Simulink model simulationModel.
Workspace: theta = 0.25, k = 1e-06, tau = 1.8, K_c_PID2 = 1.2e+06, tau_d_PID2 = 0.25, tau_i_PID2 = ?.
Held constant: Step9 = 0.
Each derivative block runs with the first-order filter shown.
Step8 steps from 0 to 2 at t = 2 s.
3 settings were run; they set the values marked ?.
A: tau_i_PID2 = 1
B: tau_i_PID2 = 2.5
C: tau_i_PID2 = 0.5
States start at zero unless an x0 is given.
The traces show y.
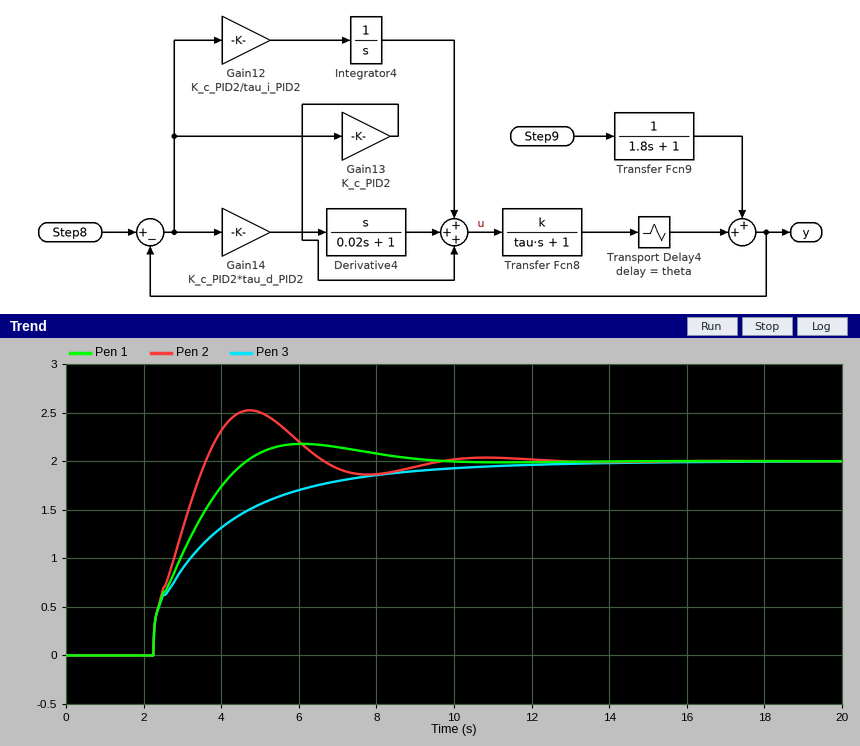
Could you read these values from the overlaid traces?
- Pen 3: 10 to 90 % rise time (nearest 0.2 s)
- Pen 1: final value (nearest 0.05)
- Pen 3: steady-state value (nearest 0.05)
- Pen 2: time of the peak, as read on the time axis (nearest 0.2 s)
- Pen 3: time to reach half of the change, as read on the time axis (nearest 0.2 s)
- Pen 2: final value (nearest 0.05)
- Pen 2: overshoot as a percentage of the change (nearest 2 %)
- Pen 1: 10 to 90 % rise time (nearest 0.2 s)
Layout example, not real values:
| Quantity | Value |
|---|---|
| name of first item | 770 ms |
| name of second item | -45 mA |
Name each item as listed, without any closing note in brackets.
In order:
| Quantity | Value |
|---|---|
| Pen 3: 10 to 90 % rise time | 4.8 s |
| Pen 1: final value | 2.00 |
| Pen 3: steady-state value | 2.00 |
| Pen 2: time of the peak, as read on the time axis | 4.8 s |
| Pen 3: time to reach half of the change, as read on the time axis | 3.2 s |
| Pen 2: final value | 2.00 |
| Pen 2: overshoot as a percentage of the change | 26 % |
| Pen 1: 10 to 90 % rise time | 1.8 s |
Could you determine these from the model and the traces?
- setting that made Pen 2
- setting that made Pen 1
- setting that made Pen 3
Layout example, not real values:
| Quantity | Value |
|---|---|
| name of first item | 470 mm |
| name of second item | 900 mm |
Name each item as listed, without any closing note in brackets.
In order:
| Quantity | Value |
|---|---|
| setting that made Pen 2 | C |
| setting that made Pen 1 | A |
| setting that made Pen 3 | B |
